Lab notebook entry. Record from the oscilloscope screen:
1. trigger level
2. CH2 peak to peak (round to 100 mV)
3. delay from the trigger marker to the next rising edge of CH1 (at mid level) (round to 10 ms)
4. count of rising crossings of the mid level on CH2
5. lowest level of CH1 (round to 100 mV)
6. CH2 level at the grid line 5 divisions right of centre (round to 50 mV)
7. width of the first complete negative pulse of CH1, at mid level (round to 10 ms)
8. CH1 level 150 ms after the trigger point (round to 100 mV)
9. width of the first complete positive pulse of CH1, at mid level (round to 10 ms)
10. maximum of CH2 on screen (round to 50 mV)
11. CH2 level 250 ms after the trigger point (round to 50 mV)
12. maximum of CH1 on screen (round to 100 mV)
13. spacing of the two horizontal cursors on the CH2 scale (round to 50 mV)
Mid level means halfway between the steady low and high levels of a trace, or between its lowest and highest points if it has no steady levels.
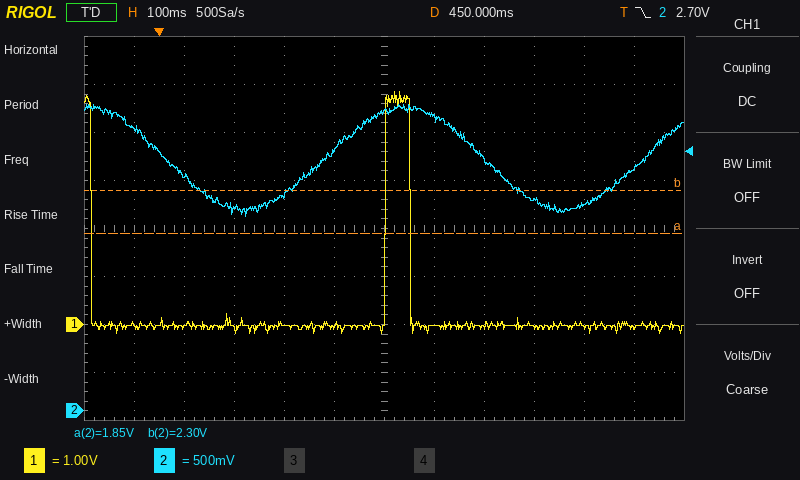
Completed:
2.70 V
1.20 V
450 ms
2
-200 mV
2.55 V
590 ms
-100 mV
50 ms
3.20 V
2.25 V
4.9 V
450 mV
